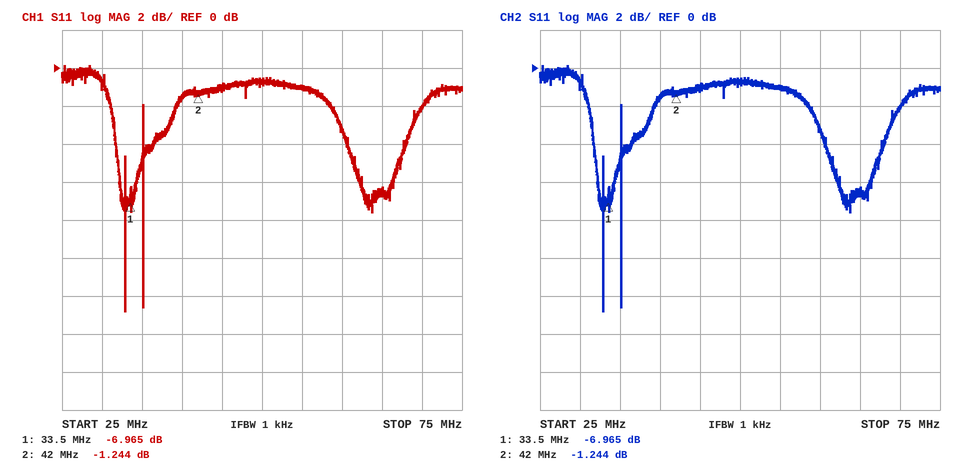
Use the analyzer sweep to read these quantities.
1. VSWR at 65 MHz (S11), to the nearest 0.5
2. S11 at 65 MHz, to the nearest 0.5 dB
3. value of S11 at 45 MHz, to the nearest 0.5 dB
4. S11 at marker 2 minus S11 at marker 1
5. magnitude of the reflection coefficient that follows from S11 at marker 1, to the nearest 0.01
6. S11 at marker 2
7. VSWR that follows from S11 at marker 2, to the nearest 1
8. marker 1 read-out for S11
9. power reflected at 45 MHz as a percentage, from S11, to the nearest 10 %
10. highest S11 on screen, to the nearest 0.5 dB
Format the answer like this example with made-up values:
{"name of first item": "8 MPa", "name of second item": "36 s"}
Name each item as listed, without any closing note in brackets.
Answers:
{"VSWR at 65 MHz (S11), to the nearest 0.5": "3.0", "S11 at 65 MHz, to the nearest 0.5 dB": "-6.5 dB", "value of S11 at 45 MHz, to the nearest 0.5 dB": "-1.0 dB", "S11 at marker 2 minus S11 at marker 1": "5.721 dB", "magnitude of the reflection coefficient that follows from S11 at marker 1, to the nearest 0.01": "0.45", "S11 at marker 2": "-1.244 dB", "VSWR that follows from S11 at marker 2, to the nearest 1": "14", "marker 1 read-out for S11": "-6.965 dB", "power reflected at 45 MHz as a percentage, from S11, to the nearest 10 %": "80 %", "highest S11 on screen, to the nearest 0.5 dB": "0.0 dB"}
